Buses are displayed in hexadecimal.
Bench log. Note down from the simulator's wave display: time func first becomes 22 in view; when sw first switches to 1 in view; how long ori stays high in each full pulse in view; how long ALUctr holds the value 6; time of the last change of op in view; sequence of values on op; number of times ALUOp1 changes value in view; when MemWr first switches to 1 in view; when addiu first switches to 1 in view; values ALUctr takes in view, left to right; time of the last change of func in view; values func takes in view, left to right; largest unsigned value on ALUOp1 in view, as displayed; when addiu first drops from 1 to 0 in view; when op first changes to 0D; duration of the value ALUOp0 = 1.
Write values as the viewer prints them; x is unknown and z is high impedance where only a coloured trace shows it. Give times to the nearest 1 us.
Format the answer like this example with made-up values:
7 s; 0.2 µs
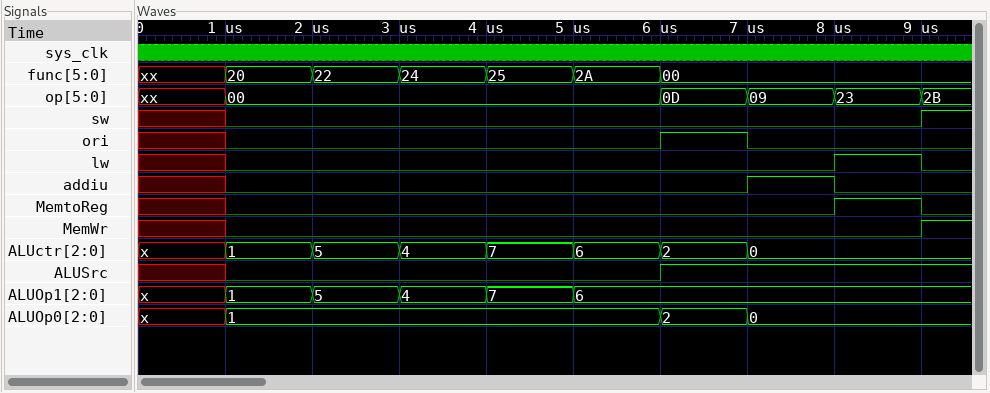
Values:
2 us; 9 us; 1 us; 1 us; 9 us; xx, 00, 0D, 09, 23, 2B; 5; 9 us; 7 us; x, 1, 5, 4, 7, 6, 2, 0; 6 us; xx, 20, 22, 24, 25, 2A, 00; 7; 8 us; 6 us; 5 us
